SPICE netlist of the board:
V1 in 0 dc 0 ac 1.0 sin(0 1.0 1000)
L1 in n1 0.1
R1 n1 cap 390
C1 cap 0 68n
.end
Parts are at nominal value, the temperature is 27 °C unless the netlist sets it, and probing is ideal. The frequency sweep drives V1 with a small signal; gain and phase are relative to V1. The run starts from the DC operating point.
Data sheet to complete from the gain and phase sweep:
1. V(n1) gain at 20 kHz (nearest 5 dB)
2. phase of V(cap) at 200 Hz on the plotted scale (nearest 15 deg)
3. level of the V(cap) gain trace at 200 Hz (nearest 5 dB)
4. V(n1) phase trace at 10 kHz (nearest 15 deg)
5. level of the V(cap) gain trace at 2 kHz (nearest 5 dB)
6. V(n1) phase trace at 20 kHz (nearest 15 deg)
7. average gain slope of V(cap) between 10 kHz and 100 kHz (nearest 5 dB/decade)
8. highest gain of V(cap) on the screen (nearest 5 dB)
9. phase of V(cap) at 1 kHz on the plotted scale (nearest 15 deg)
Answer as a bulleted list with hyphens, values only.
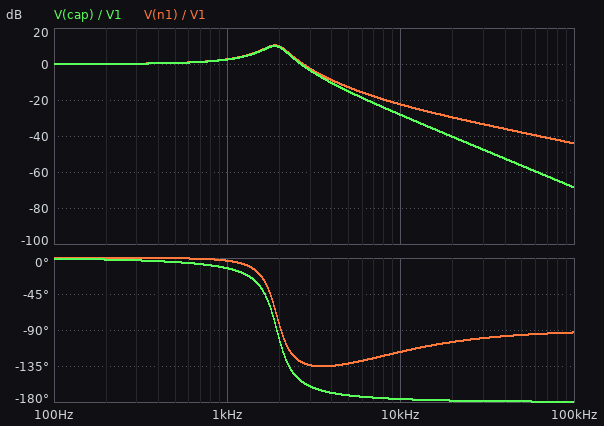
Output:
- -30 dB
- 0 deg
- 0 dB
- -120 deg
- 10 dB
- -105 deg
- -40 dB/decade
- 10 dB
- -15 deg
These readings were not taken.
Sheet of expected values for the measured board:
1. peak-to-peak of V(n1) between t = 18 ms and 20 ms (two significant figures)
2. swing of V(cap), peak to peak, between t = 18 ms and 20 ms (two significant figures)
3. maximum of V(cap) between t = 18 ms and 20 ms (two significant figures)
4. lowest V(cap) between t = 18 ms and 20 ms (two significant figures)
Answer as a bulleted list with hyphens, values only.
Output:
- 2.7 V
- 2.7 V
- 1.3 V
- -1.3 V
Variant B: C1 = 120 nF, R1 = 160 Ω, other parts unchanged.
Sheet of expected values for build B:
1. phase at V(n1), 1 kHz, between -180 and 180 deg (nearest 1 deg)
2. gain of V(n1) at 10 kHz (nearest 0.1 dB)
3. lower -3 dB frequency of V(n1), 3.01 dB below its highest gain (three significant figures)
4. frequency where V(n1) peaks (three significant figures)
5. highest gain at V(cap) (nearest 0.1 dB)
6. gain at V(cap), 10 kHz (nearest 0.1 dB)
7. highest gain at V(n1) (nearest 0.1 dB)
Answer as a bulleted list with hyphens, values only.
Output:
- -6 deg
- -29.4 dB
- 1.31 kHz
- 1.44 kHz
- 15.2 dB
- -33.3 dB
- 15.3 dB
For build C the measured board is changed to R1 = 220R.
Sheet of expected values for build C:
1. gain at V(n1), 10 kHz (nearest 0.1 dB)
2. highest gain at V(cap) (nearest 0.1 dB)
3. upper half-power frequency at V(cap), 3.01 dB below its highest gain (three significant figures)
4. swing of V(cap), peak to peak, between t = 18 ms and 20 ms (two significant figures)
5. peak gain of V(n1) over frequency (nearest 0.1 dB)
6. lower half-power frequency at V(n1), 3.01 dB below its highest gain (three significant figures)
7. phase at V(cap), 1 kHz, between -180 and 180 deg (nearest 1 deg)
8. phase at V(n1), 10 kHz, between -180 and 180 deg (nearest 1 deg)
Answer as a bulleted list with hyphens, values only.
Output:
- -25.5 dB
- 14.9 dB
- 2.08 kHz
- 2.7 V
- 15.0 dB
- 1.73 kHz
- -7 deg
- -135 deg
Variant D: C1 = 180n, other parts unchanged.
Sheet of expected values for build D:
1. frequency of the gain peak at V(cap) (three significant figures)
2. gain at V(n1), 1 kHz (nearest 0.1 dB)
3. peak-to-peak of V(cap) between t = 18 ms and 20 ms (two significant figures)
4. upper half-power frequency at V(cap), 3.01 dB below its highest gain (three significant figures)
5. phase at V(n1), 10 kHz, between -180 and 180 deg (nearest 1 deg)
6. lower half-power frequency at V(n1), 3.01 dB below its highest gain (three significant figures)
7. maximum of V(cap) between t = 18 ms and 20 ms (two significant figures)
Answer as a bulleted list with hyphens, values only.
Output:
- 1.10 kHz
- 6.3 dB
- 3.8 V
- 1.39 kHz
- -99 deg
- 762 Hz
- 1.9 V
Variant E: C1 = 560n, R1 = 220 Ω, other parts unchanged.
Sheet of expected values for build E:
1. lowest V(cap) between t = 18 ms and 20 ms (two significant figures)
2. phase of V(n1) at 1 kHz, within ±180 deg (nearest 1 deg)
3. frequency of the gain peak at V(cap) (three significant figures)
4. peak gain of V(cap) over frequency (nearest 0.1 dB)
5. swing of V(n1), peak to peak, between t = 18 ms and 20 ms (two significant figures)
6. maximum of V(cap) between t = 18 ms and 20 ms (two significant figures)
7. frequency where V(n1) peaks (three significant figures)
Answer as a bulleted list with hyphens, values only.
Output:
- -700 mV
- -110 deg
- 625 Hz
- 6.0 dB
- 1.8 V
- 700 mV
- 635 Hz
